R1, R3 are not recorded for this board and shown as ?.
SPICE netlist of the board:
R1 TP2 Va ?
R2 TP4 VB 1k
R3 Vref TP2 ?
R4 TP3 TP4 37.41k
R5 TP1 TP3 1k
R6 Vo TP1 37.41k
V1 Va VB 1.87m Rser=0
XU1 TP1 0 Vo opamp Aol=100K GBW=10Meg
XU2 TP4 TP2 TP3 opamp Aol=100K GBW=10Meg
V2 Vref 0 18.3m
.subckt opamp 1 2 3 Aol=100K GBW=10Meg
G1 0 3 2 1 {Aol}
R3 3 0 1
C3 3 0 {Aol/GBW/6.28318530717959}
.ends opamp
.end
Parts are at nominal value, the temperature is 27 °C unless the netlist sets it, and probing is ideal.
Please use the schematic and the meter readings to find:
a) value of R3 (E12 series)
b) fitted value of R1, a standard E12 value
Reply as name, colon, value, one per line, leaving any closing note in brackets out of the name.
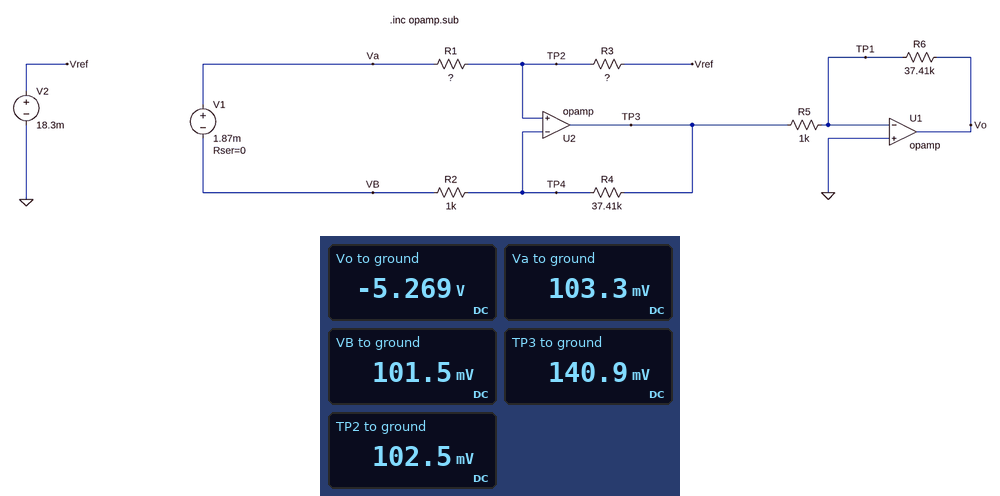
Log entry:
value of R3: 82 kΩ
fitted value of R1, a standard E12 value: 820 Ω
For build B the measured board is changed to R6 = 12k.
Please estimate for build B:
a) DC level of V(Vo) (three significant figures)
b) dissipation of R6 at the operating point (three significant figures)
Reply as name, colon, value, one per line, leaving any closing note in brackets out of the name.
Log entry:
DC level of V(Vo): -1.69 V
dissipation of R6 at the operating point: 238 µW
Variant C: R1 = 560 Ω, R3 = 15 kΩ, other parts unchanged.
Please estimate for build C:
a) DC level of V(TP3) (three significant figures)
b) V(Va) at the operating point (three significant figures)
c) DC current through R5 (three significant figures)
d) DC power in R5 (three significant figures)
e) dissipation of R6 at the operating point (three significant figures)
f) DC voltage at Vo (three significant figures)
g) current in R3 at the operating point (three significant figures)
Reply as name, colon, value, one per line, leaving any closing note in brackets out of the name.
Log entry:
DC level of V(TP3): 81.1 mV
V(Va) at the operating point: 36.9 mV
DC current through R5: 81.1 µA
DC power in R5: 6.57 µW
dissipation of R6 at the operating point: 246 µW
DC voltage at Vo: -3.03 V
current in R3 at the operating point: 1.20 µA
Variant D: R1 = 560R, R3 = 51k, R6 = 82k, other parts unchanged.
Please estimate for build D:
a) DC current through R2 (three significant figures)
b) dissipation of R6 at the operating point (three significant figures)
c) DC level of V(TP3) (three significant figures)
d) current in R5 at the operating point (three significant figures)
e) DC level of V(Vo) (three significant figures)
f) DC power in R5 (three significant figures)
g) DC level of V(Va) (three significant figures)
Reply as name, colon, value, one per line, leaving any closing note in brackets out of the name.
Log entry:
DC current through R2: 1.20 µA
dissipation of R6 at the operating point: 1.26 mW
DC level of V(TP3): 124 mV
current in R5 at the operating point: 124 µA
DC level of V(Vo): -10.2 V
DC power in R5: 15.4 µW
DC level of V(Va): 80.1 mV
